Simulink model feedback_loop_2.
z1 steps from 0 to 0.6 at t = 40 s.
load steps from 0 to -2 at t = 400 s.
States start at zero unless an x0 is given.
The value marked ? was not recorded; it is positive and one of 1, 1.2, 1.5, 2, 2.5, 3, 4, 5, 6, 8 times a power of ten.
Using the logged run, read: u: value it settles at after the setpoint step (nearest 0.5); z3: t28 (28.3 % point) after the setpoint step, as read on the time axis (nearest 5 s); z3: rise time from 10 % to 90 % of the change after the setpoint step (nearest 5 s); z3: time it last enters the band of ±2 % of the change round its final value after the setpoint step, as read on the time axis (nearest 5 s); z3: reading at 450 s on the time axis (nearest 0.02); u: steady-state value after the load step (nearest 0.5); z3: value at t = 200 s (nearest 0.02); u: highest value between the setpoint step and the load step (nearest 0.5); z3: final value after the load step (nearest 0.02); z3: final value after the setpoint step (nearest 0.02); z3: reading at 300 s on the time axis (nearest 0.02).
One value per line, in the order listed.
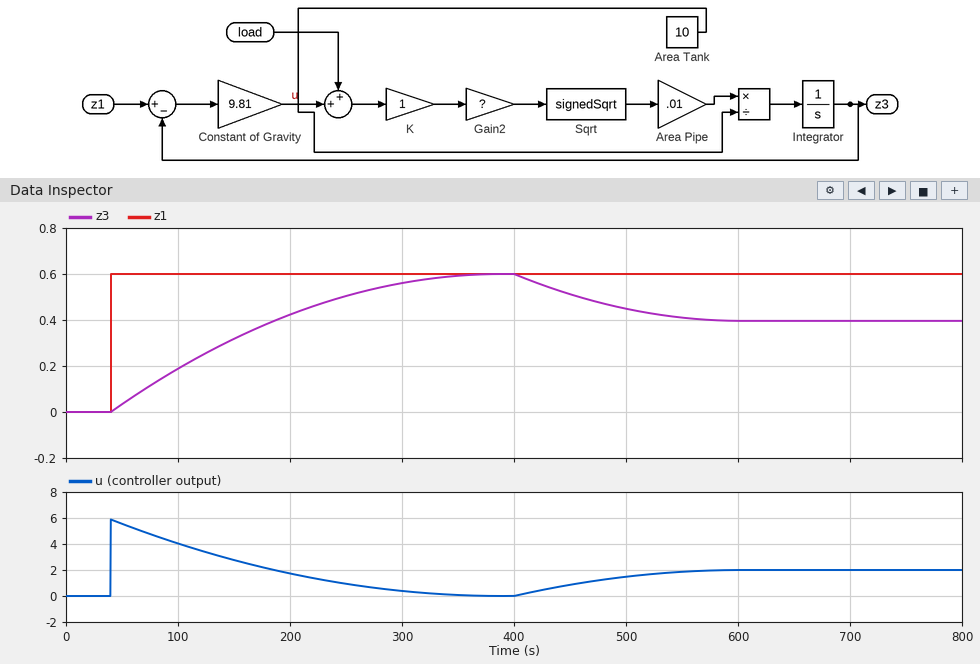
0.0
95 s
220 s
340 s
0.52
2.0
0.42
6.0
0.40
0.60
0.56
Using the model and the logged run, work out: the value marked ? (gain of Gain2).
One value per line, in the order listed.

2
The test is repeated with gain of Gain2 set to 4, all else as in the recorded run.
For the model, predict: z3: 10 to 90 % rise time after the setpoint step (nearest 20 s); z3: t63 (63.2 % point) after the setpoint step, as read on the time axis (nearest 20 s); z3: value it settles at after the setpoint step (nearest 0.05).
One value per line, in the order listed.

160 s
140 s
0.60
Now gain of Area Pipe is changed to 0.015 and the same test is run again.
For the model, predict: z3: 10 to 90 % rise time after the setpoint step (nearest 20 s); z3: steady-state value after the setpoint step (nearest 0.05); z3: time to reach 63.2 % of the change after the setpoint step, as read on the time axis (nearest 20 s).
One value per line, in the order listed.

140 s
0.60
140 s
